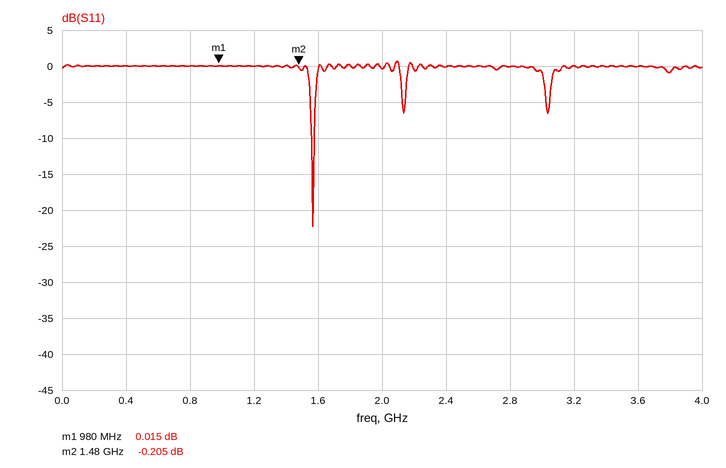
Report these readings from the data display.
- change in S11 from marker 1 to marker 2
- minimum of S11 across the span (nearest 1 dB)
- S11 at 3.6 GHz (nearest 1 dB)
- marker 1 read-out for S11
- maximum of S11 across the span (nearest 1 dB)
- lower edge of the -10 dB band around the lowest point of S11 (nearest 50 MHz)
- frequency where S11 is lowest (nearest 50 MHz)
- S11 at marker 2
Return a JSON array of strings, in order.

["-0.220 dB", "-22 dB", "0 dB", "0.015 dB", "1 dB", "1.55 GHz", "1.55 GHz", "-0.205 dB"]
